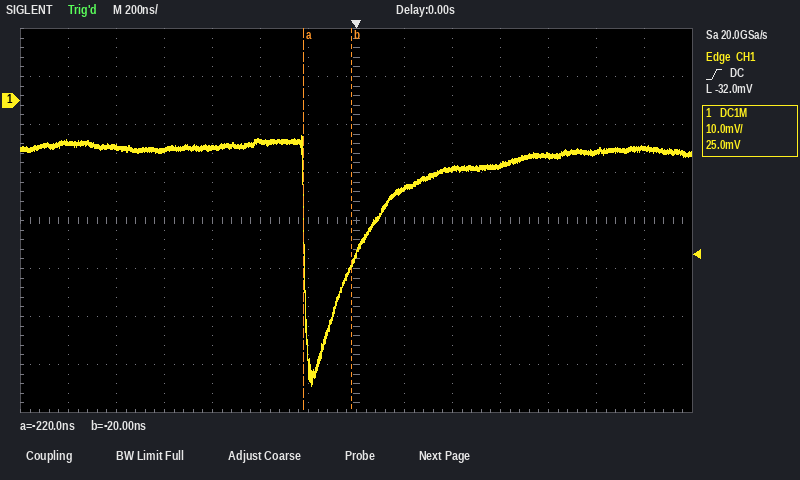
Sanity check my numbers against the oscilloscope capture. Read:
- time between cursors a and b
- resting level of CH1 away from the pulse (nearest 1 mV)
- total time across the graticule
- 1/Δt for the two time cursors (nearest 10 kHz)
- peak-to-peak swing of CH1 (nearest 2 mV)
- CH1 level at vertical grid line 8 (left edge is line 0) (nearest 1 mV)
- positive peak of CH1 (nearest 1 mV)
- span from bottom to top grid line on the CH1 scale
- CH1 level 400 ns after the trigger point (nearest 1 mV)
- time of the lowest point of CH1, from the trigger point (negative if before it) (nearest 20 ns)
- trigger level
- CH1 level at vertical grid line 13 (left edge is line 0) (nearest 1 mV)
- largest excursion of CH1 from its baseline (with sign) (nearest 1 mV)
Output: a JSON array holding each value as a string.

["200 ns", "-10 mV", "2.8 µs", "5.00 MHz", "52 mV", "-18 mV", "-7 mV", "80 mV", "-14 mV", "-180 ns", "-32.0 mV", "-10 mV", "-49 mV"]
